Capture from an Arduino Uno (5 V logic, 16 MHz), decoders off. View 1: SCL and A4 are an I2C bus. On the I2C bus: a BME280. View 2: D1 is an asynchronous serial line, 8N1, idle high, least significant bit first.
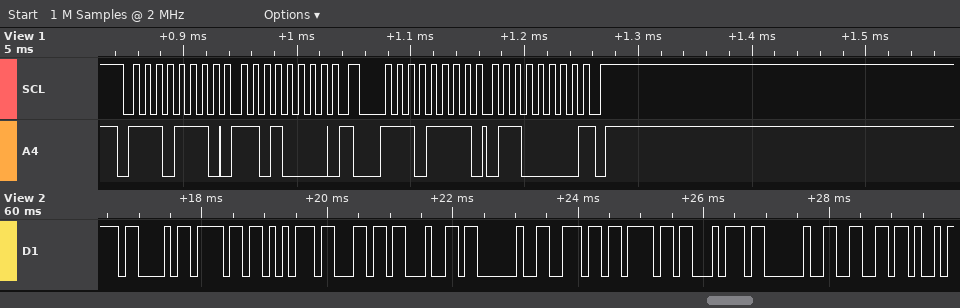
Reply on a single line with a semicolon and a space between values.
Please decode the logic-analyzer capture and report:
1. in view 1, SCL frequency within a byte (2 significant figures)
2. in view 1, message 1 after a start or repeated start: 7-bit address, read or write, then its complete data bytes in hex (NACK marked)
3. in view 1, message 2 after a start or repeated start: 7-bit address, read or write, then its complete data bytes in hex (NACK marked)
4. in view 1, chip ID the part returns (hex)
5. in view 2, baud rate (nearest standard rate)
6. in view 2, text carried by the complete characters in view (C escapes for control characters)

100 kHz; 0x77 write: D0; 0x77 read: 60 NACK; 0x60; 9600 baud; "Could not f"
